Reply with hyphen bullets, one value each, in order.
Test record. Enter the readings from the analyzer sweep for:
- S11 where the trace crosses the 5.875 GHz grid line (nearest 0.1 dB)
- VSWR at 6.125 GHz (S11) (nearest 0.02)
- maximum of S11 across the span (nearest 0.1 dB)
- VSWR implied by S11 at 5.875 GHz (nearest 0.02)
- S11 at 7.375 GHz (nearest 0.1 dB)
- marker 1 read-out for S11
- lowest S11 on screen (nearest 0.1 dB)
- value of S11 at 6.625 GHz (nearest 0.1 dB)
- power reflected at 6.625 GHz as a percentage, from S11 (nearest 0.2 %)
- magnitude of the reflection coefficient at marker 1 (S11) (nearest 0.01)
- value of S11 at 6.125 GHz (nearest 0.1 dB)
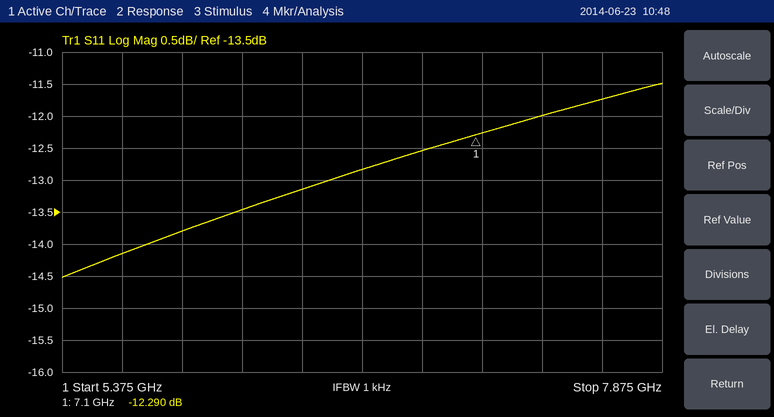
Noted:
- -13.8 dB
- 1.54
- -11.5 dB
- 1.52
- -12.0 dB
- -12.290 dB
- -14.5 dB
- -12.8 dB
- 5.2 %
- 0.24
- -13.5 dB
